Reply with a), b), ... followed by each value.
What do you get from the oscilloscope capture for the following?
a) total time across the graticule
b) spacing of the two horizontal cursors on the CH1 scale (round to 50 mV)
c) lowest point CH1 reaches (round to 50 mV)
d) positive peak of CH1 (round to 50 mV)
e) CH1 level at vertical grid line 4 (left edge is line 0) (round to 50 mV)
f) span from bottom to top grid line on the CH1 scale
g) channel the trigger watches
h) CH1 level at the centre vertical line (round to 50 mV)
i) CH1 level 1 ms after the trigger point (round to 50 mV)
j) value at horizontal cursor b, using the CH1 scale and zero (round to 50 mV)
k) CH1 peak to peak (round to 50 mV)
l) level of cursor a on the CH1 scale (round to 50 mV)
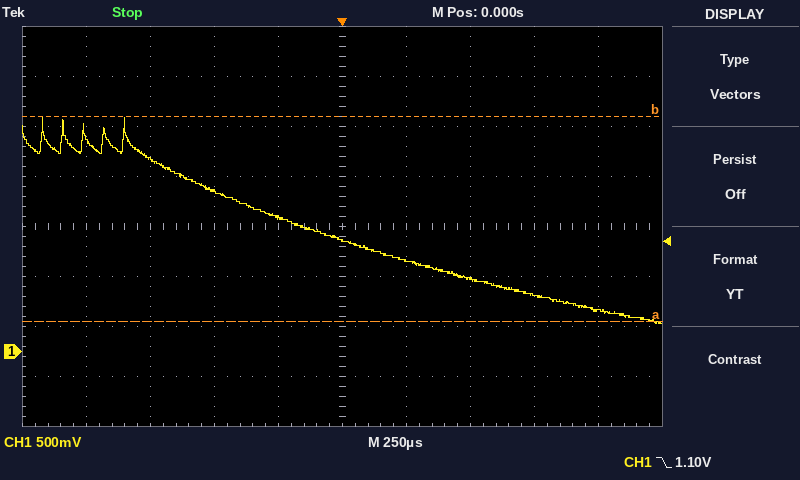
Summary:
a) 2.5 ms
b) 2.05 V
c) 300 mV
d) 2.35 V
e) 1.35 V
f) 4 V
g) CH1
h) 1.10 V
i) 400 mV
j) 2.35 V
k) 2.05 V
l) 300 mV
